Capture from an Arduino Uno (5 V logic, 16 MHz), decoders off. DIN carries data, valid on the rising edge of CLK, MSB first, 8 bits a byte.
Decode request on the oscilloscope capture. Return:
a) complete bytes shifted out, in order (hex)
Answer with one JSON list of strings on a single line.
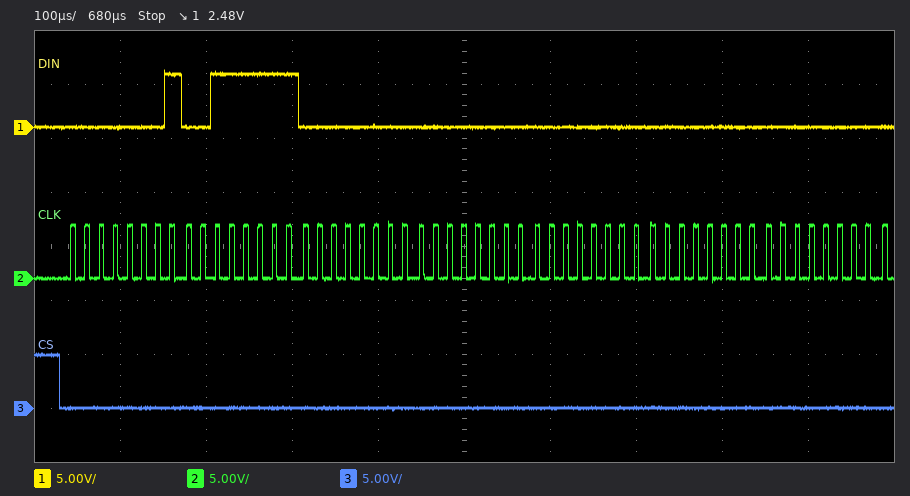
["01 3F 00 00 00 00 00"]
